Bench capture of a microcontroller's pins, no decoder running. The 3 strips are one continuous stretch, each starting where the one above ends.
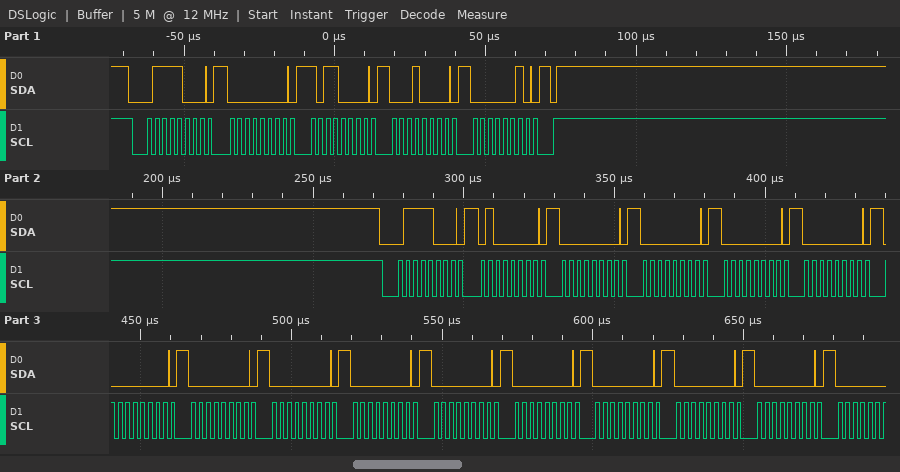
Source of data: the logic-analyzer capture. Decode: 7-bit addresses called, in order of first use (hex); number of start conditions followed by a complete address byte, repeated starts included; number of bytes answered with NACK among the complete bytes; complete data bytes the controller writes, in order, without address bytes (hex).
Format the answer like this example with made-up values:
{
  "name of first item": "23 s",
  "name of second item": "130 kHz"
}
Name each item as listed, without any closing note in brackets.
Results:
{
  "7-bit addresses called, in order of first use": "0x3C",
  "number of start conditions followed by a complete address byte, repeated starts included": "2",
  "number of bytes answered with NACK among the complete bytes": "0",
  "complete data bytes the controller writes, in order, without address bytes": "00 B0 10 02 40 00 00 00 00 00 00 00 00 00 00 00 00 00"
}
